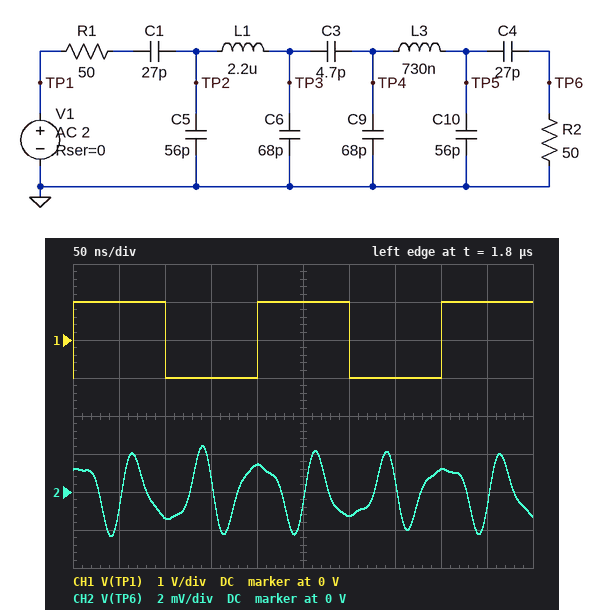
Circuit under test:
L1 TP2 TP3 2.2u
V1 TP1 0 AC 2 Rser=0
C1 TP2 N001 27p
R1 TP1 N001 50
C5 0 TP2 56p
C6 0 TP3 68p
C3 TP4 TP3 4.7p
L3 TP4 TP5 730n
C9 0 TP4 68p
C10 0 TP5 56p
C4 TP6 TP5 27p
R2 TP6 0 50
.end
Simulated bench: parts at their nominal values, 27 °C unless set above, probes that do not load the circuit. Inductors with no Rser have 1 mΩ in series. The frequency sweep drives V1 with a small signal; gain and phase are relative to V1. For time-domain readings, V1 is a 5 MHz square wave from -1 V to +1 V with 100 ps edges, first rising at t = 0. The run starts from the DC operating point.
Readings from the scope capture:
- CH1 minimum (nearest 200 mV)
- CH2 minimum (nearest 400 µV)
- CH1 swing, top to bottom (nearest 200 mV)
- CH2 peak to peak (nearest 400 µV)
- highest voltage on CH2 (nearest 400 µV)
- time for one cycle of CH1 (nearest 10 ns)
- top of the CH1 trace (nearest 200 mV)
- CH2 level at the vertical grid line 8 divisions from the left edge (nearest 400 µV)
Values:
-1.0 V
-2.4 mV
2.0 V
4.8 mV
2.4 mV
200 ns
1.0 V
1.2 mV
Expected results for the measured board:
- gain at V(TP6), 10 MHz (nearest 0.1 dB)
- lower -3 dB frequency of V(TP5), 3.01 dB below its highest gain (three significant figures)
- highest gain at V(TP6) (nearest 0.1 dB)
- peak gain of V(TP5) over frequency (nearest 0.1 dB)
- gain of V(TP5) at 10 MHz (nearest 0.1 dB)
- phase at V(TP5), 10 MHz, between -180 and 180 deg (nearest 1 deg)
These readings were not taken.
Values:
-62.5 dB
17.1 MHz
-25.8 dB
-9.0 dB
-41.0 dB
-4 deg
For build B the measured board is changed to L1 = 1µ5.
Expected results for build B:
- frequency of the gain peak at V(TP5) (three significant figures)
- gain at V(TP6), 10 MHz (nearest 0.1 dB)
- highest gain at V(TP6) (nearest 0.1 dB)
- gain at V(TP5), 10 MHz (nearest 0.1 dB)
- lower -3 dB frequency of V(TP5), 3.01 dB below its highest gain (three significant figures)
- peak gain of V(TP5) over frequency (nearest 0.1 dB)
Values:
20.9 MHz
-63.8 dB
-23.5 dB
-42.3 dB
20.6 MHz
-8.4 dB
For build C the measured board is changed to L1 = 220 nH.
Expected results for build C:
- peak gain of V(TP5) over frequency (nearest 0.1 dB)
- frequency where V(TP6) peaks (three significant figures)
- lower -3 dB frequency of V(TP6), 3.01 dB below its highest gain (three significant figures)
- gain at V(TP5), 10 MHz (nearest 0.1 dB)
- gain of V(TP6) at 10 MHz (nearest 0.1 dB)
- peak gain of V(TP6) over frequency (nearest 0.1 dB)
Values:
-14.1 dB
30.0 MHz
29.5 MHz
-44.3 dB
-65.8 dB
-26.2 dB
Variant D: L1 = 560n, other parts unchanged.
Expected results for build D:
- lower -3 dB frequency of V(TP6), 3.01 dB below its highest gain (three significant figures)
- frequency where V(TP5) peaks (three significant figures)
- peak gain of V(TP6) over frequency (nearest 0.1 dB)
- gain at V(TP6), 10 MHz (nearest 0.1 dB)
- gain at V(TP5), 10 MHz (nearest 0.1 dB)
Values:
29.5 MHz
30.0 MHz
-17.0 dB
-65.3 dB
-43.8 dB
